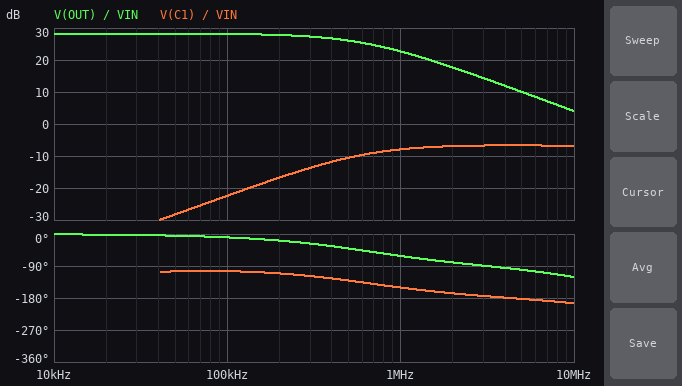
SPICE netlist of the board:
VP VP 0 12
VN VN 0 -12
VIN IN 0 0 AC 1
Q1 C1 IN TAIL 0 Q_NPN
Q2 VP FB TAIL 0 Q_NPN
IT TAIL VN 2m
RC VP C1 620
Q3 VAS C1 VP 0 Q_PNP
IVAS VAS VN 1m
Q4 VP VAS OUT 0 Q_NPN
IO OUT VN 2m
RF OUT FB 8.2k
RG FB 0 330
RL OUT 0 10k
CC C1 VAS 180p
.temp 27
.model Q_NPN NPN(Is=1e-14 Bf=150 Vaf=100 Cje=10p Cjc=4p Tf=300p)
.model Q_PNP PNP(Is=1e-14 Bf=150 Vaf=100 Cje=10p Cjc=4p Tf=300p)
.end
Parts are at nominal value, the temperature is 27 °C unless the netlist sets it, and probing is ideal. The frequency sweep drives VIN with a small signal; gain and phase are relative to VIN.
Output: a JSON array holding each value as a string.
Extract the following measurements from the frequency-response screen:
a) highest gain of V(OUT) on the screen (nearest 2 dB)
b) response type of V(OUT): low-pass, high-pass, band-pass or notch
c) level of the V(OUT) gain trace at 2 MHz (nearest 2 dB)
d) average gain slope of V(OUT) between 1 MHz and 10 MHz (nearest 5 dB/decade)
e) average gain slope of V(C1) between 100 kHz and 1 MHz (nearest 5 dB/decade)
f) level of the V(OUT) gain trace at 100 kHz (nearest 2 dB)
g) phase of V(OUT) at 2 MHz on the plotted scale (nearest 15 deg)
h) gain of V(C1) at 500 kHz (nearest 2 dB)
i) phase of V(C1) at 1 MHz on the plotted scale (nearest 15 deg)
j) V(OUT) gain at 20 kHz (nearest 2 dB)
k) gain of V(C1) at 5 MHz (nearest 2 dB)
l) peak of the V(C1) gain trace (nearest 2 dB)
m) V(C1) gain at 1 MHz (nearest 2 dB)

["28 dB", "low-pass", "18 dB", "-20 dB/decade", "15 dB/decade", "28 dB", "-75 deg", "-10 dB", "-150 deg", "28 dB", "-6 dB", "-6 dB", "-8 dB"]
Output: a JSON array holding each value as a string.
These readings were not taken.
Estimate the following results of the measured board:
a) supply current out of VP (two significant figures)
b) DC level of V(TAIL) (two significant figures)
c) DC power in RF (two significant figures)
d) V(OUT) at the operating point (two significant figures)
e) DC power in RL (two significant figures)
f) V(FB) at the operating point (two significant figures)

["5.0 mA", "-650 mV", "220 nW", "-46 mV", "210 nW", "-3.5 mV"]
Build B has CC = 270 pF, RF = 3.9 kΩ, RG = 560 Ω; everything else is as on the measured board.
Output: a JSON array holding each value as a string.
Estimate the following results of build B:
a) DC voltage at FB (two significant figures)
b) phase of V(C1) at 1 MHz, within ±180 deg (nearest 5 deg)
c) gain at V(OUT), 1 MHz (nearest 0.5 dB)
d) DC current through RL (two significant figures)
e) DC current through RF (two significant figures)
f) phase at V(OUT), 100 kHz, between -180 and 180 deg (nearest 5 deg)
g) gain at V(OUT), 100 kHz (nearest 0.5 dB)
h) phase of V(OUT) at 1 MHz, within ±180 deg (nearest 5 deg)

["-3.5 mV", "-130 deg", "16.5 dB", "660 nA", "780 nA", "-5 deg", "18.0 dB", "-40 deg"]
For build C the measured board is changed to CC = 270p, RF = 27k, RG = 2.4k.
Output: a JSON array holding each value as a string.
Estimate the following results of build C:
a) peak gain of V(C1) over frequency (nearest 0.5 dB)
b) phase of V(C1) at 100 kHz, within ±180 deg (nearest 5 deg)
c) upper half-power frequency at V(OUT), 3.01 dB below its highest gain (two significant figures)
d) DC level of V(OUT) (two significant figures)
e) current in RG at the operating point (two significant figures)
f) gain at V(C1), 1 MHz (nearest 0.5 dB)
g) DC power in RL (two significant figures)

["-8.0 dB", "-100 deg", "830 kHz", "110 mV", "1.5 µA", "-9.5 dB", "1.1 µW"]
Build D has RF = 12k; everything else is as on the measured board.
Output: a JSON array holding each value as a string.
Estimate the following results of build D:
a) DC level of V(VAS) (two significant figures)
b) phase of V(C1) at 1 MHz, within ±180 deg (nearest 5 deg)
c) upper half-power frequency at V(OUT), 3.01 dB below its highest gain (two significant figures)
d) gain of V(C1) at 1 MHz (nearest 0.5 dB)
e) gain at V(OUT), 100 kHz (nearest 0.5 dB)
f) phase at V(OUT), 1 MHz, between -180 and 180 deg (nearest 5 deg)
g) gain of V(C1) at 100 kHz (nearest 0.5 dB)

["600 mV", "-160 deg", "420 kHz", "-7.5 dB", "31.0 dB", "-70 deg", "-19.5 dB"]
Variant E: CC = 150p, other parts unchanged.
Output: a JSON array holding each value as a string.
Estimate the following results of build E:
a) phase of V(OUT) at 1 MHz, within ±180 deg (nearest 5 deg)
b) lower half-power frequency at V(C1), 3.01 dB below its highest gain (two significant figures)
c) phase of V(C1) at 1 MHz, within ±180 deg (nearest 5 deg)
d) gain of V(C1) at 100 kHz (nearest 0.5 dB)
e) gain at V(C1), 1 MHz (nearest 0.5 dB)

["-55 deg", "710 kHz", "-145 deg", "-24.0 dB", "-8.5 dB"]
